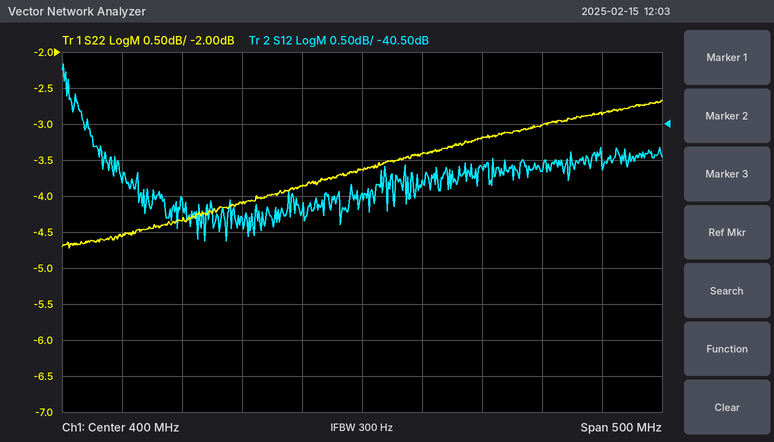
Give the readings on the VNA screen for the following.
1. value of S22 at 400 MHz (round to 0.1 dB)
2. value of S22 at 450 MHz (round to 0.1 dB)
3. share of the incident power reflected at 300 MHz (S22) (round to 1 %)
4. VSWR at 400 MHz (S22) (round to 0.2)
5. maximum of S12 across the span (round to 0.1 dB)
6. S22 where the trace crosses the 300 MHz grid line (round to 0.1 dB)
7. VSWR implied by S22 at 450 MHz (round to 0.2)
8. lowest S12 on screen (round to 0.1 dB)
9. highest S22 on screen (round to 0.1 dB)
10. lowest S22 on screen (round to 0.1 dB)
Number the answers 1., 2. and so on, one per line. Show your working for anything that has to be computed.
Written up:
1. -3.6 dB
2. -3.4 dB
3. 10^(-4.1/10) ≈ 39 %
4. |Γ| = 10^(-3.6/20) = 0.6607; VSWR = (1 + 0.6607)/(1 − 0.6607) ≈ 4.89, so 4.8 to the nearest 0.2
5. -39.7 dB
6. -4.1 dB
7. |Γ| = 10^(-3.4/20) = 0.6761; VSWR = (1 + 0.6761)/(1 − 0.6761) ≈ 5.2
8. -42.1 dB
9. -2.7 dB
10. -4.7 dB
